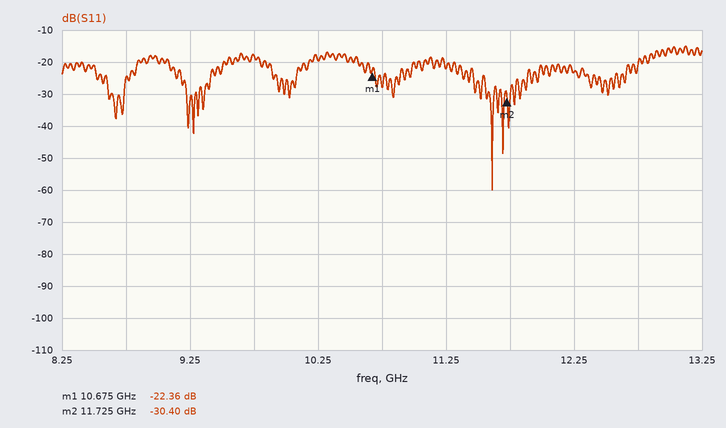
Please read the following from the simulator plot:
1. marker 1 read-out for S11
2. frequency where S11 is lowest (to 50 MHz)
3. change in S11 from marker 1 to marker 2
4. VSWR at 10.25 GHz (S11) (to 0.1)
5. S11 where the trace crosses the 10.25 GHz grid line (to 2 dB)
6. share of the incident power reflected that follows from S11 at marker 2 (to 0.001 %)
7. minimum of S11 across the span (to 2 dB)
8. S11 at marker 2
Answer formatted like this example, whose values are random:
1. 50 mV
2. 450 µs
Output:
1. -22.36 dB
2. 11.60 GHz
3. -8.04 dB
4. 1.2
5. -20 dB
6. 0.091 %
7. -60 dB
8. -30.40 dB
